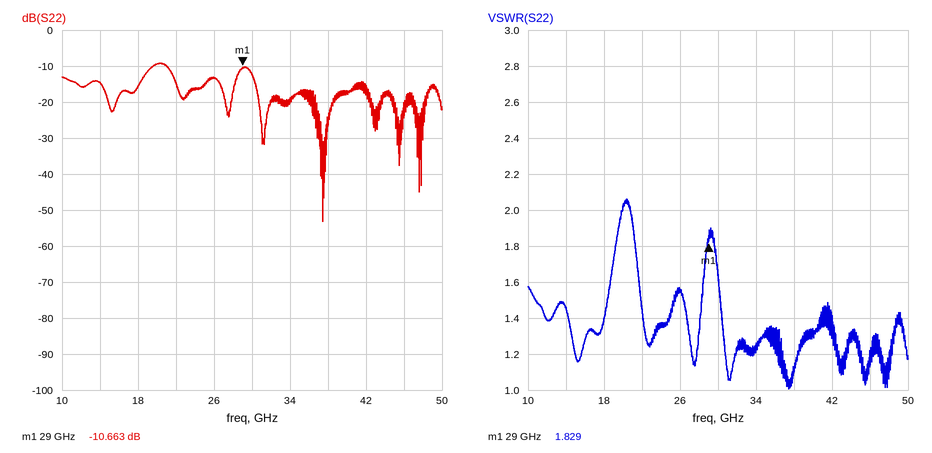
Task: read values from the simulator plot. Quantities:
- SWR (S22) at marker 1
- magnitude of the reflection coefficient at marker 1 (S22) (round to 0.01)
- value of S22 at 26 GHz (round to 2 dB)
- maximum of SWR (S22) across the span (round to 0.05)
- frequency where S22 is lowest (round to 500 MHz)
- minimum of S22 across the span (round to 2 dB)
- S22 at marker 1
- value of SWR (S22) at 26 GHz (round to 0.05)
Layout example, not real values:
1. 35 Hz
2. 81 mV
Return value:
1. 1.829
2. 0.29
3. -14 dB
4. 2.05
5. 37.5 GHz
6. -54 dB
7. -10.663 dB
8. 1.55
